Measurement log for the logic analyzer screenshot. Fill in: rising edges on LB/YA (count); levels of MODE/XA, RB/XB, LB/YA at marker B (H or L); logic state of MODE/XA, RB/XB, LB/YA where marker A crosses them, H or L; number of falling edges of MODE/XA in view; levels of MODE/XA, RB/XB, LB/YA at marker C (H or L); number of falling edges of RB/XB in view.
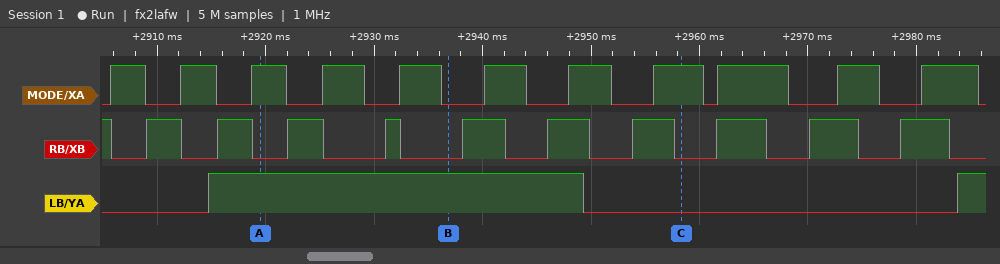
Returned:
2
MODE/XA=L, RB/XB=L, LB/YA=H
MODE/XA=H, RB/XB=L, LB/YA=H
11
MODE/XA=H, RB/XB=L, LB/YA=L
11
